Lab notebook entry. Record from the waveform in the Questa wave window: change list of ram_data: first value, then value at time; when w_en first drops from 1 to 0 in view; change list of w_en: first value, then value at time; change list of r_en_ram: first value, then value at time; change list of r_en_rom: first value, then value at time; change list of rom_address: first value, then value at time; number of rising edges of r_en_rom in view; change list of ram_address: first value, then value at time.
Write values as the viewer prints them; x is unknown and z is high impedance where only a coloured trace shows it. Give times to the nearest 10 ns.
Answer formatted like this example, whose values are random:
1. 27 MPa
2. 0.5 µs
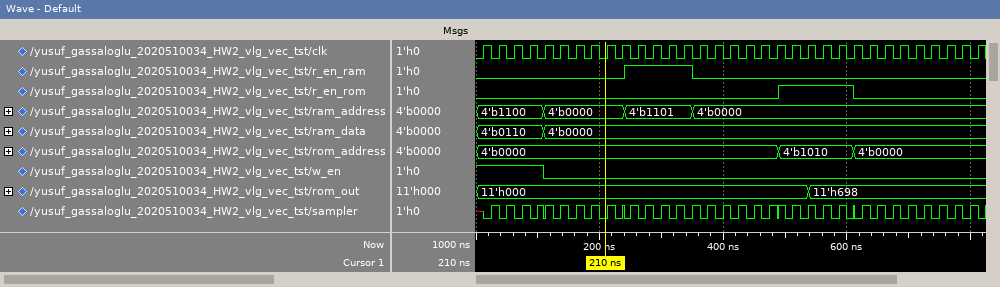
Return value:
1. 4'b0110, 4'b0000 at 110 ns
2. 110 ns
3. 1, 0 at 110 ns
4. 0, 1 at 240 ns, 0 at 350 ns
5. 0, 1 at 490 ns, 0 at 610 ns
6. 4'b0000, 4'b1010 at 490 ns, 4'b0000 at 610 ns
7. 1
8. 4'b1100, 4'b0000 at 110 ns, 4'b1101 at 240 ns, 4'b0000 at 350 ns
